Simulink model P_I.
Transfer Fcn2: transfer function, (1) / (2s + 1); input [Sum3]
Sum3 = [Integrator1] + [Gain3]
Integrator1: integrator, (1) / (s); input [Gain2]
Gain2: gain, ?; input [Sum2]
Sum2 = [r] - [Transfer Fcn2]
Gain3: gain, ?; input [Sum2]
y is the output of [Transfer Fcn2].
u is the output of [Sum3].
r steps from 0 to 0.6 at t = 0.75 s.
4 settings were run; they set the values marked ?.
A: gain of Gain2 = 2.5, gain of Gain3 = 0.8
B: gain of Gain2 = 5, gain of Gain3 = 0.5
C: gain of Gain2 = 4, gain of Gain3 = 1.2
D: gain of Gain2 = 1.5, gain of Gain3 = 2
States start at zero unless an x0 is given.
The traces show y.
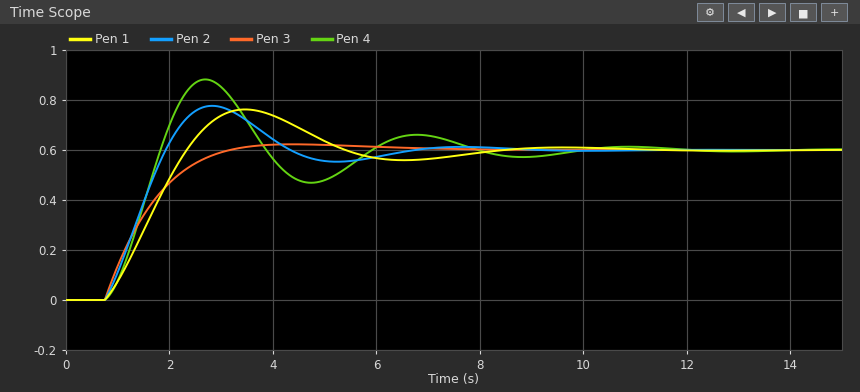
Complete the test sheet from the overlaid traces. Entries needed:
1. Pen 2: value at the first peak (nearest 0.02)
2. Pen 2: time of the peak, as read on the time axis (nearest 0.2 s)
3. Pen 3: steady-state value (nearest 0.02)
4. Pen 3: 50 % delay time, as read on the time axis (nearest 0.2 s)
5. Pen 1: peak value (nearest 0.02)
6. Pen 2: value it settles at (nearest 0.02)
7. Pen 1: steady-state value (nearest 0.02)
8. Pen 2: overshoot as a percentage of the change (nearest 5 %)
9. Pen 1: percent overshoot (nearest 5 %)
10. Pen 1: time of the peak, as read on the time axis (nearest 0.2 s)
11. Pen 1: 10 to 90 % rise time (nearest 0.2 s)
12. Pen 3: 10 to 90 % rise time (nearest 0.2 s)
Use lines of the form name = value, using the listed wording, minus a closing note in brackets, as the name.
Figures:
Pen 2: value at the first peak = 0.78
Pen 2: time of the peak, as read on the time axis = 2.8 s
Pen 3: steady-state value = 0.60
Pen 3: 50 % delay time, as read on the time axis = 1.4 s
Pen 1: peak value = 0.76
Pen 2: value it settles at = 0.60
Pen 1: steady-state value = 0.60
Pen 2: overshoot as a percentage of the change = 30 %
Pen 1: percent overshoot = 25 %
Pen 1: time of the peak, as read on the time axis = 3.4 s
Pen 1: 10 to 90 % rise time = 1.2 s
Pen 3: 10 to 90 % rise time = 1.6 s
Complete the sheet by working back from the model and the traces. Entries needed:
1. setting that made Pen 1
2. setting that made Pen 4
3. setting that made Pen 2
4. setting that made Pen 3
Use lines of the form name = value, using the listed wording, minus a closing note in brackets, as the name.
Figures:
setting that made Pen 1 = A
setting that made Pen 4 = B
setting that made Pen 2 = C
setting that made Pen 3 = D
